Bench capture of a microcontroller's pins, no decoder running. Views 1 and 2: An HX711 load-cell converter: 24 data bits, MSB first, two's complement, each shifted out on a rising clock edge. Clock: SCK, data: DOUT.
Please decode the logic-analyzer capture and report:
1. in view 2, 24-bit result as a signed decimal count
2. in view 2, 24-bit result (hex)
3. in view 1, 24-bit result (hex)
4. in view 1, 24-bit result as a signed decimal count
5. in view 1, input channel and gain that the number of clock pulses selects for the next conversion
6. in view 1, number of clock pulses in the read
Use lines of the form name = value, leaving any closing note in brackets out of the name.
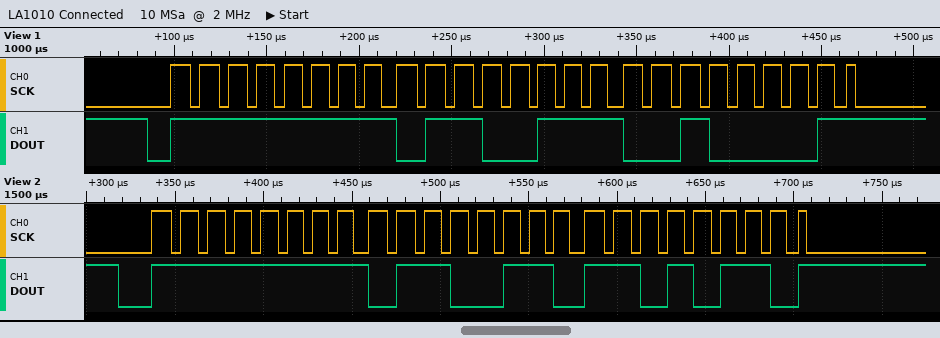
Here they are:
in view 2, 24-bit result as a signed decimal count = -39210
in view 2, 24-bit result = 0xFF66D6
in view 1, 24-bit result = 0xFF6721
in view 1, 24-bit result as a signed decimal count = -39135
in view 1, input channel and gain that the number of clock pulses selects for the next conversion = channel A, gain 128
in view 1, number of clock pulses in the read = 25
